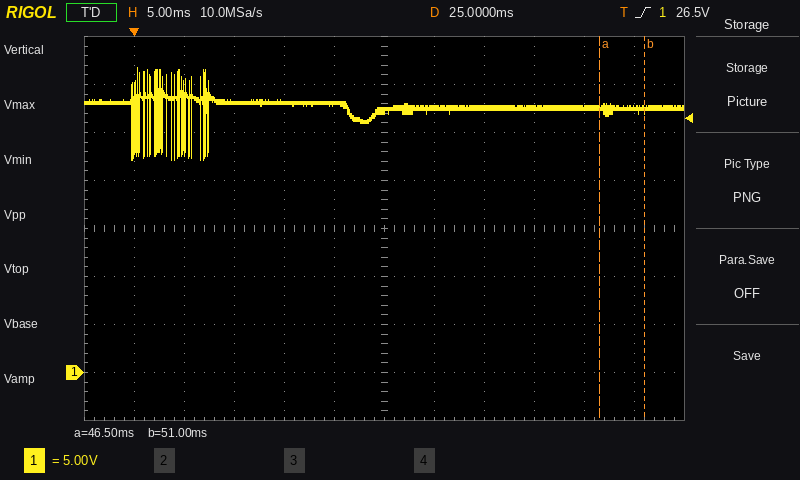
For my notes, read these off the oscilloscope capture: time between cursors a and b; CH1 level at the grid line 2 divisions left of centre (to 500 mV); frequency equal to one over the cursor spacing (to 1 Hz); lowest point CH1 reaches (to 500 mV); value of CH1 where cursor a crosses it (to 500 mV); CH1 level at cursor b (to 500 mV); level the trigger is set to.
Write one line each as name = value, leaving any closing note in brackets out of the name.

time between cursors a and b = 4.5 ms
CH1 level at the grid line 2 divisions left of centre = 28.0 V
frequency equal to one over the cursor spacing = 222 Hz
lowest point CH1 reaches = 22.0 V
value of CH1 where cursor a crosses it = 27.5 V
CH1 level at cursor b = 27.5 V
level the trigger is set to = 26.5 V
